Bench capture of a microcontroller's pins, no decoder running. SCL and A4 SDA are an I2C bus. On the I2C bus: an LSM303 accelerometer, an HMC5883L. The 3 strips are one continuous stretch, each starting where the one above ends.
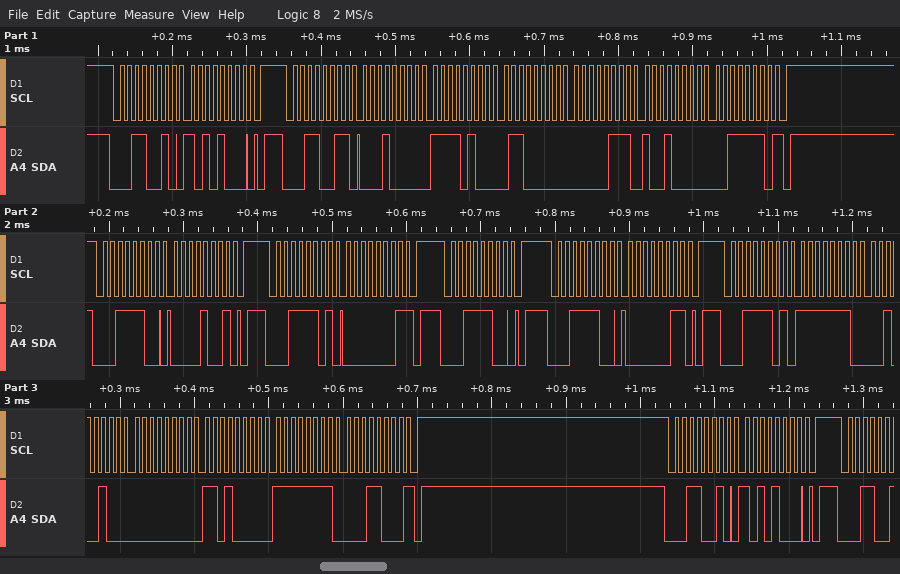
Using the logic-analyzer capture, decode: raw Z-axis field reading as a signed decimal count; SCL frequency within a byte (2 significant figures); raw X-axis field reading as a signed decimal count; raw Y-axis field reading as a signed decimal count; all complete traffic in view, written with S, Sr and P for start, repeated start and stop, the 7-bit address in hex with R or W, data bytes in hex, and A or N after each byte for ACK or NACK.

208
100 kHz
-476
-232
S 19W A A8 A P S 19R A 10 A F4 A 60 A 07 A 90 A 3E N P S 1EW A 09 A P S 1ER A 01 N P S 1EW A P S 1EW A 03 A P S 1ER A FE A 24 A 00 A D0 A FF A 18 N P S 19W A A8 A P
